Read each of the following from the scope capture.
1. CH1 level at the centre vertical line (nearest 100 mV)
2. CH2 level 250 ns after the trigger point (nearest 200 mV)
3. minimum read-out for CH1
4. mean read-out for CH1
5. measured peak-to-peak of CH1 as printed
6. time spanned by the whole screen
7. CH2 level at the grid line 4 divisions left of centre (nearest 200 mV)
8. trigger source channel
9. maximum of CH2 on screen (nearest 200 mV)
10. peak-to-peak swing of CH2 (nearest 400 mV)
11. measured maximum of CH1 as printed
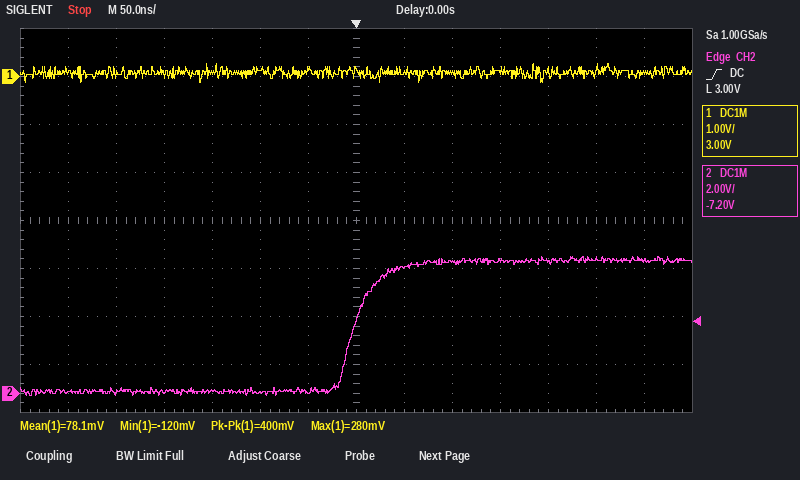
100 mV
5.6 V
-120 mV
78.1 mV
400 mV
700 ns
0.0 V
CH2
5.6 V
5.6 V
280 mV
